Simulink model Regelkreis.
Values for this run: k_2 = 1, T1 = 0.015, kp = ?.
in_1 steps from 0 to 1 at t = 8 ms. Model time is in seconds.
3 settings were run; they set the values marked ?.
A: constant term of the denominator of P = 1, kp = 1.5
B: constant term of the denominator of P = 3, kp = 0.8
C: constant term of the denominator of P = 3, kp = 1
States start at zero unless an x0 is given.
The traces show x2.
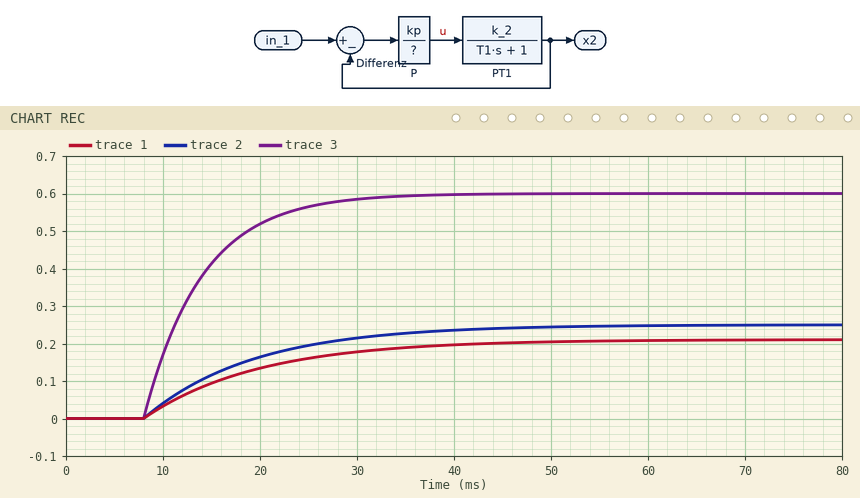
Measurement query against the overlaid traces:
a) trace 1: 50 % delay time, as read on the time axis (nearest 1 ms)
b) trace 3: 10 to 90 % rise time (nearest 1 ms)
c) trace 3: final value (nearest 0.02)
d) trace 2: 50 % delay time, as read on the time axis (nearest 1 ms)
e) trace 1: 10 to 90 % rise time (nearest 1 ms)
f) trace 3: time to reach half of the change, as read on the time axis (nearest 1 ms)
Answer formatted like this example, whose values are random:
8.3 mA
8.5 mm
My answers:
16 ms
13 ms
0.60
16 ms
26 ms
12 ms
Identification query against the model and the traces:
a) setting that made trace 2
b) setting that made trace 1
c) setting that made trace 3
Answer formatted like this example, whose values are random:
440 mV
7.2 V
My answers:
C
B
A
